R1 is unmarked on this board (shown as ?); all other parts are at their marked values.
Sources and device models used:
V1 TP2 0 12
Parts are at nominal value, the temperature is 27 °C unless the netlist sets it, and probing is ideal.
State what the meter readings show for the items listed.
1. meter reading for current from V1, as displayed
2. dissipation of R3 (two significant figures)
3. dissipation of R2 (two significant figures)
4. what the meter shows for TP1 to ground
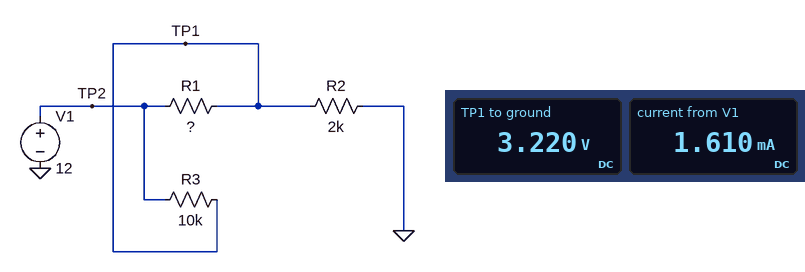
1.610 mA
7.7 mW
5.2 mW
3.220 V
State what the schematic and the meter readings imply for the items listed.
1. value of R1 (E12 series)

12 kΩ
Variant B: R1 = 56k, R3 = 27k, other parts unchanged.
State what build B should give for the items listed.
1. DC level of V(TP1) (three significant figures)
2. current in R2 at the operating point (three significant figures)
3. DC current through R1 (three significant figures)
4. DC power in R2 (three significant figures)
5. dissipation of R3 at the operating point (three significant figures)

1.19 V
594 µA
193 µA
705 µW
4.33 mW
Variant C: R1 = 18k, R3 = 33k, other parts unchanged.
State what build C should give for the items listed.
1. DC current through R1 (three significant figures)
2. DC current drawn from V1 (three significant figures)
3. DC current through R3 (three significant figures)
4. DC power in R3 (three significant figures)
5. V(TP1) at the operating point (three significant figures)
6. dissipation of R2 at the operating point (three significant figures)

569 µA
879 µA
310 µA
3.18 mW
1.76 V
1.55 mW
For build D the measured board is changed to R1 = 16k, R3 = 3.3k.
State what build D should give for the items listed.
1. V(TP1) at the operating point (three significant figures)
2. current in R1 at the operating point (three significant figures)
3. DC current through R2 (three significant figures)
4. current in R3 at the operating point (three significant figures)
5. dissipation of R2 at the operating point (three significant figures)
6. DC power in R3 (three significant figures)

5.07 V
433 µA
2.53 mA
2.10 mA
12.8 mW
14.6 mW
